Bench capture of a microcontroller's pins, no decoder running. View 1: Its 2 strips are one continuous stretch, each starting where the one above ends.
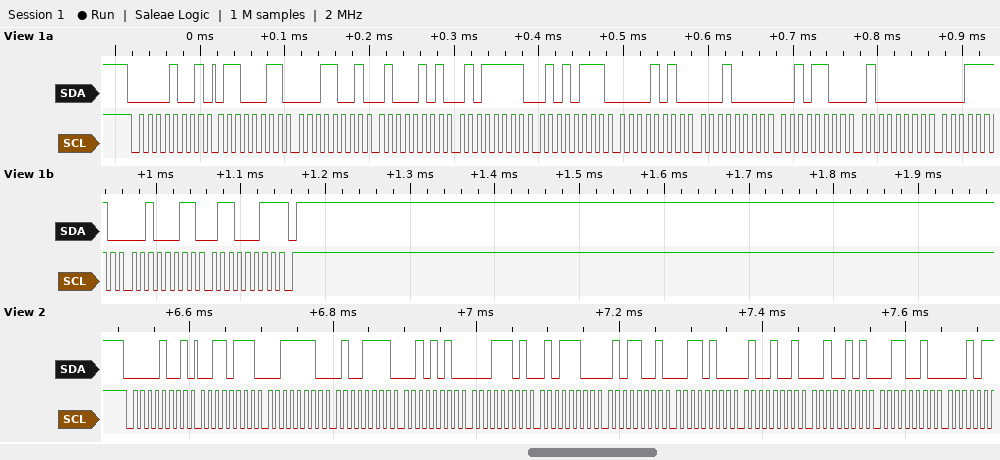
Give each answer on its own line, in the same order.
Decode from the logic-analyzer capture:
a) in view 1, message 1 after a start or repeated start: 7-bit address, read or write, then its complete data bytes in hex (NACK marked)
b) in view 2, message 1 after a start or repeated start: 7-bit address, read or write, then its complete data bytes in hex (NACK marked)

0x04 read: 63 19 45 5F 57 0A 10 2C 40 1E 23 63 NACK
0x04 read: 37 3E 4F 2A 1D 5C 59 34 49 25 32
